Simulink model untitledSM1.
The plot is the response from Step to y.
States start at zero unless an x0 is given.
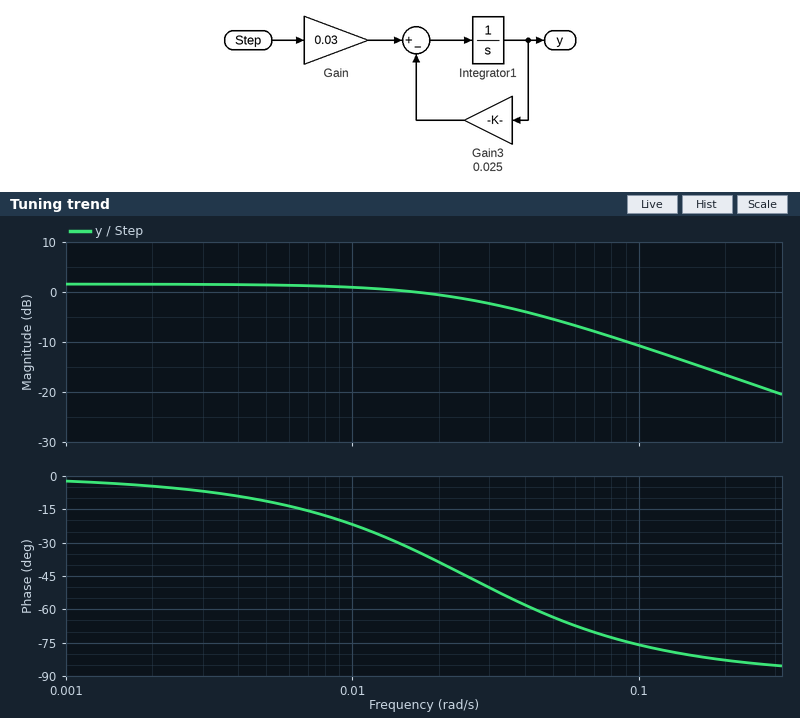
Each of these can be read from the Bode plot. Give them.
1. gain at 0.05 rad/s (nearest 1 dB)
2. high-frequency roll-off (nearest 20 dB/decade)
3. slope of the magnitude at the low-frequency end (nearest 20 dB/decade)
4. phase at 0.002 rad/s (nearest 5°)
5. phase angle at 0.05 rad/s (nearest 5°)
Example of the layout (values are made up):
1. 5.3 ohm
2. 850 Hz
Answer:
1. -5 dB
2. -20 dB/decade
3. 0 dB/decade
4. -5°
5. -65°
